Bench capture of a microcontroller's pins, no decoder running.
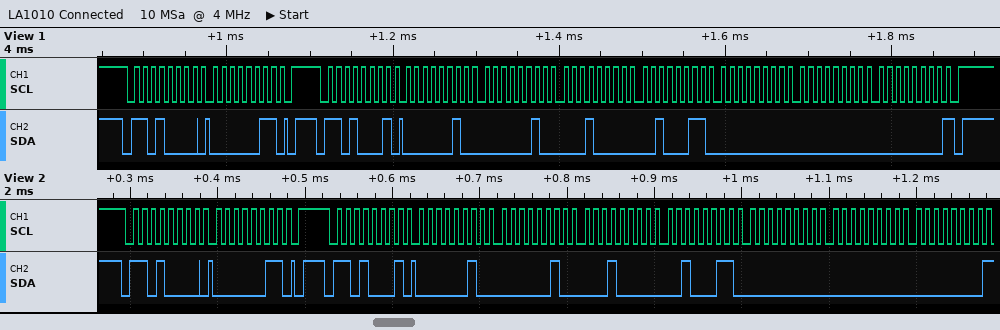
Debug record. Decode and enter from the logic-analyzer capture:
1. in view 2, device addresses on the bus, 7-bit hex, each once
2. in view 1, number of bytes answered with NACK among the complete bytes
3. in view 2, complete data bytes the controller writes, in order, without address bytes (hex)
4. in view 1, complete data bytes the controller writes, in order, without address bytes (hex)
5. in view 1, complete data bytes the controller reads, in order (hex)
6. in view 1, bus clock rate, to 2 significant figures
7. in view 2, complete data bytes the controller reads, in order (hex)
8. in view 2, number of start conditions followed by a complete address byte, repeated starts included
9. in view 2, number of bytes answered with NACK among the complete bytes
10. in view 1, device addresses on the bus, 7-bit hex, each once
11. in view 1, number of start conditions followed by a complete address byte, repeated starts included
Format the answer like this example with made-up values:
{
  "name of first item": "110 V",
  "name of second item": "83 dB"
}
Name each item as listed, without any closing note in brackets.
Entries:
{
  "in view 2, device addresses on the bus, 7-bit hex, each once": "0x68",
  "in view 1, number of bytes answered with NACK among the complete bytes": "1",
  "in view 2, complete data bytes the controller writes, in order, without address bytes": "03",
  "in view 1, complete data bytes the controller writes, in order, without address bytes": "03",
  "in view 1, complete data bytes the controller reads, in order": "02 02 10 23 00 00 00",
  "in view 1, bus clock rate, to 2 significant figures": "100 kHz",
  "in view 2, complete data bytes the controller reads, in order": "02 02 10 23 00 00 00",
  "in view 2, number of start conditions followed by a complete address byte, repeated starts included": "2",
  "in view 2, number of bytes answered with NACK among the complete bytes": "1",
  "in view 1, device addresses on the bus, 7-bit hex, each once": "0x68",
  "in view 1, number of start conditions followed by a complete address byte, repeated starts included": "2"
}
